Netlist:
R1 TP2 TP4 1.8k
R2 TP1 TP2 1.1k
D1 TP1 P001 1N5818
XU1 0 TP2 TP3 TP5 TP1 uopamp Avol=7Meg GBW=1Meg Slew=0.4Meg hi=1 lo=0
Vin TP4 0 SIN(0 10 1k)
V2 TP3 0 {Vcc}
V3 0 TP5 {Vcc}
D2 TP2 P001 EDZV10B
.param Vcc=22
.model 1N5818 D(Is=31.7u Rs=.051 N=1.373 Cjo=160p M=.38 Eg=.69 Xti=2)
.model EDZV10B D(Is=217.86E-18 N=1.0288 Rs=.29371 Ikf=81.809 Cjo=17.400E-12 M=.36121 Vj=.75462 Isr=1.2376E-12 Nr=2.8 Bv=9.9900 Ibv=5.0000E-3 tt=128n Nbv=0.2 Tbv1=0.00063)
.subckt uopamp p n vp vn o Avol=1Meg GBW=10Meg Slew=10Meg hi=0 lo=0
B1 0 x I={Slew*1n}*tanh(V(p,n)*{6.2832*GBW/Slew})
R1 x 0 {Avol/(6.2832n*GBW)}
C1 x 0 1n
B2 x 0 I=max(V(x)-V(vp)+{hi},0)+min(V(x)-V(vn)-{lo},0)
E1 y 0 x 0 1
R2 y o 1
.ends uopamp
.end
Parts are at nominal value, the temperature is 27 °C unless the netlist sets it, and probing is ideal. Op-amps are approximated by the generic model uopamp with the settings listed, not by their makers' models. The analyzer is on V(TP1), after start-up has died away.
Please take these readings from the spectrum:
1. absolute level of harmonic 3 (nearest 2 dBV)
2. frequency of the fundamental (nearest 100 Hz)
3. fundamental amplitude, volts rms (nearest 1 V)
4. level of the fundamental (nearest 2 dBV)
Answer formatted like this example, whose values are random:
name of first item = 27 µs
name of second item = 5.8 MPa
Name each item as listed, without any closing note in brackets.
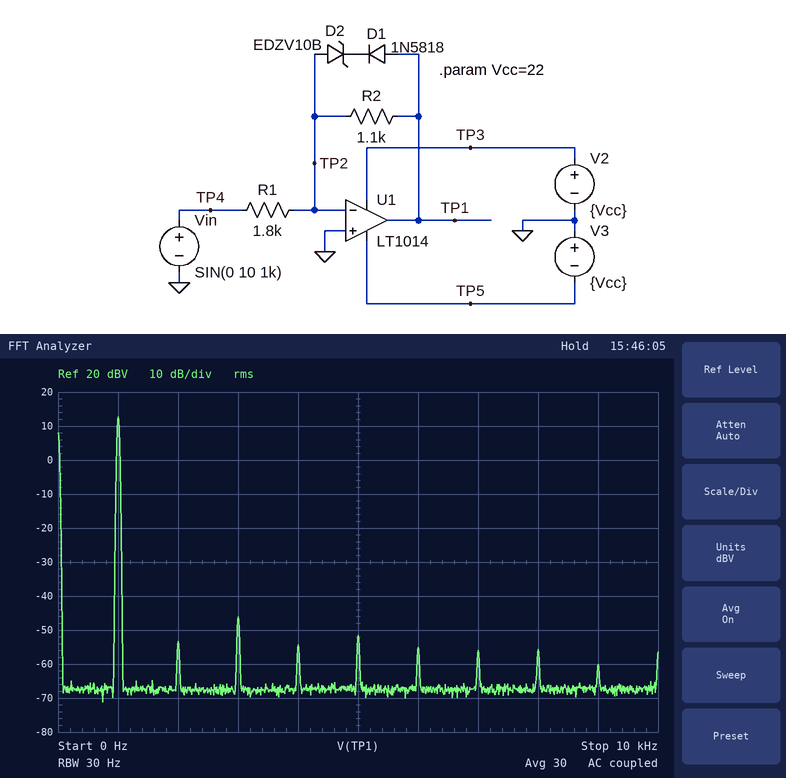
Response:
absolute level of harmonic 3 = -46 dBV
frequency of the fundamental = 1.0 kHz
fundamental amplitude, volts rms = 4 V
level of the fundamental = 12 dBV
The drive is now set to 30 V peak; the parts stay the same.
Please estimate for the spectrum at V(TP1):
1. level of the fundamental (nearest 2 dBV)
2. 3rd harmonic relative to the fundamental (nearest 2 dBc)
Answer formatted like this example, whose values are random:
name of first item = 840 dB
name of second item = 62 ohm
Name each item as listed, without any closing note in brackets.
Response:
level of the fundamental = 20 dBV
3rd harmonic relative to the fundamental = -22 dBc
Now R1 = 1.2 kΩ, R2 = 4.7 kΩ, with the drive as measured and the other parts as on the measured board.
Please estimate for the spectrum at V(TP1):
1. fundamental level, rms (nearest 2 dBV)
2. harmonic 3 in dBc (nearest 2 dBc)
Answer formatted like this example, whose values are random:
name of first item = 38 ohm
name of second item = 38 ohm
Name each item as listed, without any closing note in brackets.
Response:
fundamental level, rms = 22 dBV
harmonic 3 in dBc = -12 dBc
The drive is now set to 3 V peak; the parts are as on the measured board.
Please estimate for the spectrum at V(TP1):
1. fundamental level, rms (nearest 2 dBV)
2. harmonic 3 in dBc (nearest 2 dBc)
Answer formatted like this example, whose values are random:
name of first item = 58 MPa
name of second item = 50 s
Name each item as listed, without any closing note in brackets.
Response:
fundamental level, rms = 2 dBV
harmonic 3 in dBc = -56 dBc
